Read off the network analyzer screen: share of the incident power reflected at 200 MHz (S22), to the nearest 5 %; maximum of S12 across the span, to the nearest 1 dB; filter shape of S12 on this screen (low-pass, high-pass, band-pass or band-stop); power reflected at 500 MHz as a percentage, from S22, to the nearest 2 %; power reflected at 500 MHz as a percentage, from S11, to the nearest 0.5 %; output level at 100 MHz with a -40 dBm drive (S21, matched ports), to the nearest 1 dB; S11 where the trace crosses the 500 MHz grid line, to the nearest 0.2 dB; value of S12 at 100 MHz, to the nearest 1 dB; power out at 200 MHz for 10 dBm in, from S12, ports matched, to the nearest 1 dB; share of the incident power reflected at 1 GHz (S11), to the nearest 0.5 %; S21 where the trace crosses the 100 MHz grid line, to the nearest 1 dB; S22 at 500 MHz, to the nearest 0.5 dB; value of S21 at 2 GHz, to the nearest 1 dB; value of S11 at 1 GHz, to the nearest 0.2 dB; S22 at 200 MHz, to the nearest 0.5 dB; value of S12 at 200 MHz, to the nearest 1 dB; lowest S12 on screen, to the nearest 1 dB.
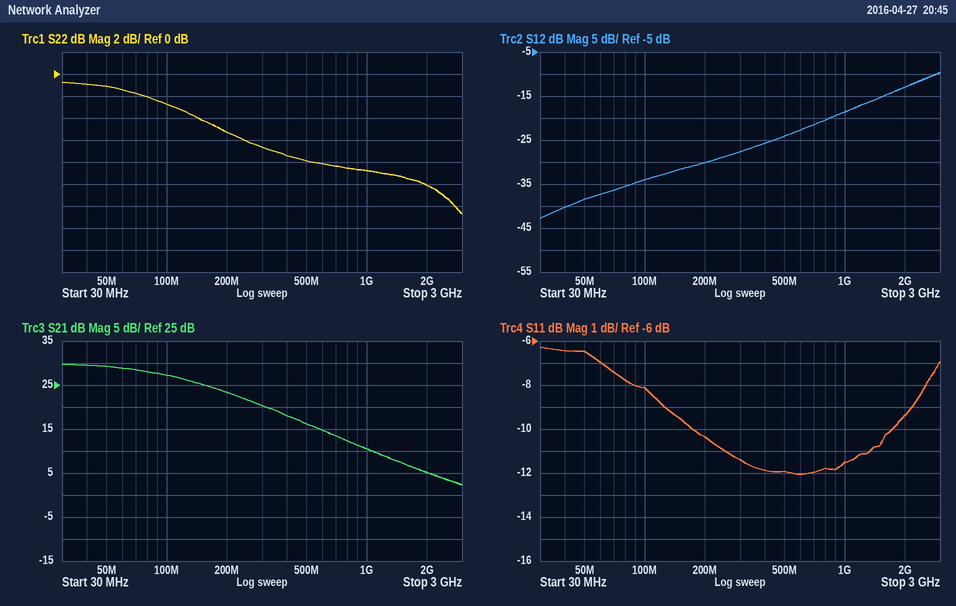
30 %
-10 dB
high-pass
16 %
6.5 %
-13 dBm
-12.0 dB
-34 dB
-20 dBm
7.0 %
27 dB
-8.0 dB
5 dB
-11.6 dB
-5.5 dB
-30 dB
-43 dB
